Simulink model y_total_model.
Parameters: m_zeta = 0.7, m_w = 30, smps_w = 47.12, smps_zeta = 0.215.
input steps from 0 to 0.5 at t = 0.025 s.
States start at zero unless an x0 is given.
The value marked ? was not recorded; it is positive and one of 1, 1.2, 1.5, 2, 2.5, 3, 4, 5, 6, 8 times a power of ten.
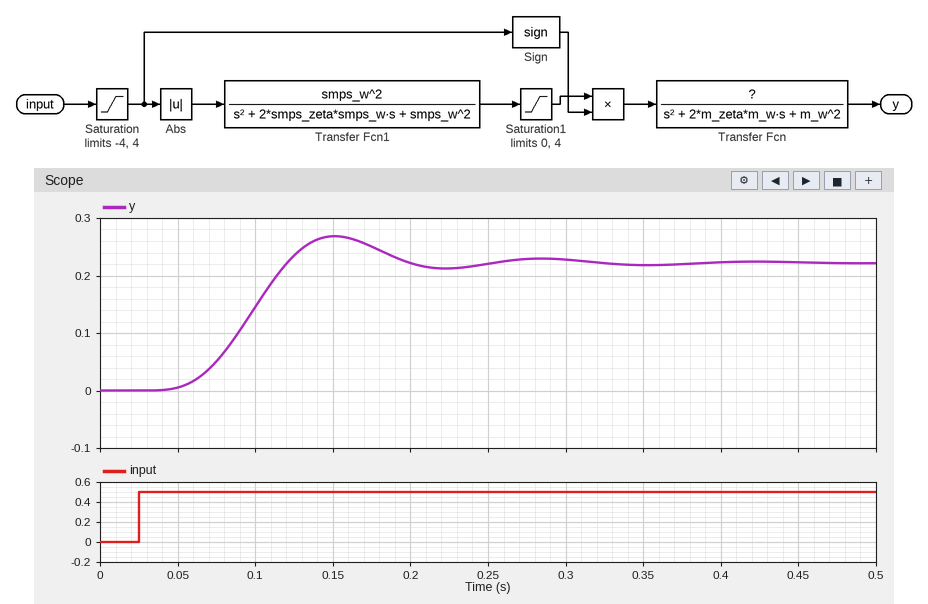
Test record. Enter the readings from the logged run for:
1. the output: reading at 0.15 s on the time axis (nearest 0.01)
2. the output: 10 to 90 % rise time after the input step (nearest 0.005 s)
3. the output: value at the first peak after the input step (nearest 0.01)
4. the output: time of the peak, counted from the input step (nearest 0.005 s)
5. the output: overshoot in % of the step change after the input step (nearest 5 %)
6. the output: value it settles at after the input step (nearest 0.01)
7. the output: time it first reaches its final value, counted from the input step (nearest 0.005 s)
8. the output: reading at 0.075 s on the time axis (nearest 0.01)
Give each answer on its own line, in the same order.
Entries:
0.27
0.050 s
0.27
0.125 s
20 %
0.22
0.095 s
0.05
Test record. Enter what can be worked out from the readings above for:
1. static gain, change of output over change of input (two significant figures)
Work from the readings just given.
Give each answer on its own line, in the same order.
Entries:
0.44
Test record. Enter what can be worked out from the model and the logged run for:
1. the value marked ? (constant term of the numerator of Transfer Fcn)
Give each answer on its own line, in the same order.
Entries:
400
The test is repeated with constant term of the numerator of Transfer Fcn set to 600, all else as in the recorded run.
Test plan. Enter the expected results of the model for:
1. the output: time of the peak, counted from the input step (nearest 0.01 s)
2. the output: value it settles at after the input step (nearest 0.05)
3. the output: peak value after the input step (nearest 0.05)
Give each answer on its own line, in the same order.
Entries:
0.13 s
0.35
0.40
